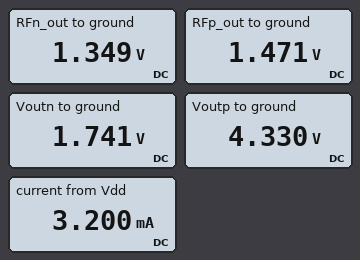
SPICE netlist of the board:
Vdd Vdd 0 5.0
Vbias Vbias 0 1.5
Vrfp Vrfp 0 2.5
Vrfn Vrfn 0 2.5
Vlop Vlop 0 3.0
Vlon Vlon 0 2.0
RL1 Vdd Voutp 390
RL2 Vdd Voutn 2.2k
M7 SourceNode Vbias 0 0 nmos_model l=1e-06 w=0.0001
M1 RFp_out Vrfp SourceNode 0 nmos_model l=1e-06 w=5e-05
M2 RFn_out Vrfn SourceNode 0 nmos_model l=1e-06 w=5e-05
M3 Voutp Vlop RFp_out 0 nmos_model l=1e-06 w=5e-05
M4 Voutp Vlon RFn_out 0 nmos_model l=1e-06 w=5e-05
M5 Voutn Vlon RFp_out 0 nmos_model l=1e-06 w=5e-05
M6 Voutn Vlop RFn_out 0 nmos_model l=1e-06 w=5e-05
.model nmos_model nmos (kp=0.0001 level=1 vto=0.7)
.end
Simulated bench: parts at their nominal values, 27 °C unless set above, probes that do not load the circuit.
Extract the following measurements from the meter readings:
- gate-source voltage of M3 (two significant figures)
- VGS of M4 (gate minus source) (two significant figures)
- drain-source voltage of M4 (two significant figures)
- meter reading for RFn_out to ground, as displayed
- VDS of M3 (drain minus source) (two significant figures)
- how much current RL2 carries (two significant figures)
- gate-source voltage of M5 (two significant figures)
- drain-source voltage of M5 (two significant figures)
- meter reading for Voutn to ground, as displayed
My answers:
1.5 V
650 mV
3.0 V
1.349 V
2.9 V
1.5 mA
530 mV
270 mV
1.741 V
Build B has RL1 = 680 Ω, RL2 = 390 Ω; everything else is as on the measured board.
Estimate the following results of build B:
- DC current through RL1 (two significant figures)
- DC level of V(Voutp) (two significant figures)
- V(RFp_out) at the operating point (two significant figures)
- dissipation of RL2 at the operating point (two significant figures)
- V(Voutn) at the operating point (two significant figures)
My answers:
1.6 mA
3.9 V
1.5 V
1.0 mW
4.4 V
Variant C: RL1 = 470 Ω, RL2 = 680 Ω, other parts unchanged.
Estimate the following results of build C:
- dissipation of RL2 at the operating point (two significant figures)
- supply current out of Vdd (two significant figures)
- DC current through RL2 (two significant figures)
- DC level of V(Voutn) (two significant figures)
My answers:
1.7 mW
3.2 mA
1.6 mA
3.9 V
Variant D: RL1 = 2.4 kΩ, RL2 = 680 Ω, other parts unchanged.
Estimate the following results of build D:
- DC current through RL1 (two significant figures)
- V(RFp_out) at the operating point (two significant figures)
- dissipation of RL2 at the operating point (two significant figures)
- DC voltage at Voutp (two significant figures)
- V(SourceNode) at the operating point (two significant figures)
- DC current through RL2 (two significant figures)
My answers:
1.4 mA
1.3 V
2.2 mW
1.6 V
890 mV
1.8 mA
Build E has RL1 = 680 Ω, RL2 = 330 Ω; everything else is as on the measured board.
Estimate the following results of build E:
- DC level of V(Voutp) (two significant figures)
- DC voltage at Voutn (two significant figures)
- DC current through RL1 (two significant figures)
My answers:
3.9 V
4.5 V
1.6 mA
